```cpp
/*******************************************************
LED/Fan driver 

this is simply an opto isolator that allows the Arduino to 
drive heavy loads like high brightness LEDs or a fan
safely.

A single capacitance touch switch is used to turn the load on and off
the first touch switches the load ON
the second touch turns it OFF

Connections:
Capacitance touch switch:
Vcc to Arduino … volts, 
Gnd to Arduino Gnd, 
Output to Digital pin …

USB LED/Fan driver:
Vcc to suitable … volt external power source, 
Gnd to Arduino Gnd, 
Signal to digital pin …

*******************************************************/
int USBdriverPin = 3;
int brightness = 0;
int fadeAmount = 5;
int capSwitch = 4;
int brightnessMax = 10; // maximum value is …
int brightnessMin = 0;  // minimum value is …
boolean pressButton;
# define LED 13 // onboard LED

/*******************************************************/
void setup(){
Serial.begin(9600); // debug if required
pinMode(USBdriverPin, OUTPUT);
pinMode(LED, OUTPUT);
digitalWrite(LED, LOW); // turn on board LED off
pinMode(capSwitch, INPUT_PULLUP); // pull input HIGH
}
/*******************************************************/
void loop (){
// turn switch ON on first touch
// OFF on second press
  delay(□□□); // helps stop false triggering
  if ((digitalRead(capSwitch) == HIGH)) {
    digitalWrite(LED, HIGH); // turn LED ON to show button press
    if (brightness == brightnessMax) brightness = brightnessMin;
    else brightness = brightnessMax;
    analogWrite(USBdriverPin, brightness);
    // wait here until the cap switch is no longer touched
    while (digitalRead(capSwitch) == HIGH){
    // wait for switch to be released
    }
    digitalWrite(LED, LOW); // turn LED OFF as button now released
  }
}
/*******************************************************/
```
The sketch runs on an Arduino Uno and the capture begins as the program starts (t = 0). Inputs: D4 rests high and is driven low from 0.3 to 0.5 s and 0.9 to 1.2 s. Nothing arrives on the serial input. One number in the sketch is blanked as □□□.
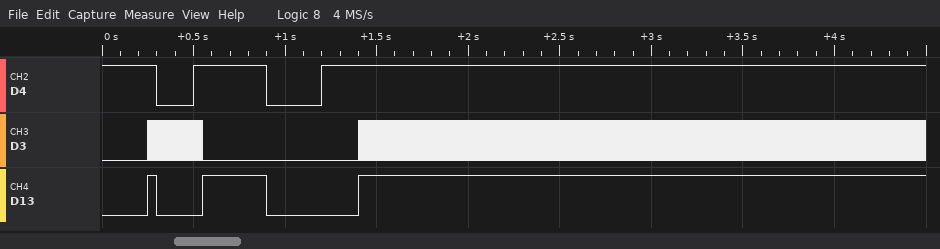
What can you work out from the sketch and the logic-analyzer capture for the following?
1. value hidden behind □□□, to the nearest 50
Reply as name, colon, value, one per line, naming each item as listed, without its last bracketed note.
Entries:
value hidden behind □□□, to the nearest 50: 250
